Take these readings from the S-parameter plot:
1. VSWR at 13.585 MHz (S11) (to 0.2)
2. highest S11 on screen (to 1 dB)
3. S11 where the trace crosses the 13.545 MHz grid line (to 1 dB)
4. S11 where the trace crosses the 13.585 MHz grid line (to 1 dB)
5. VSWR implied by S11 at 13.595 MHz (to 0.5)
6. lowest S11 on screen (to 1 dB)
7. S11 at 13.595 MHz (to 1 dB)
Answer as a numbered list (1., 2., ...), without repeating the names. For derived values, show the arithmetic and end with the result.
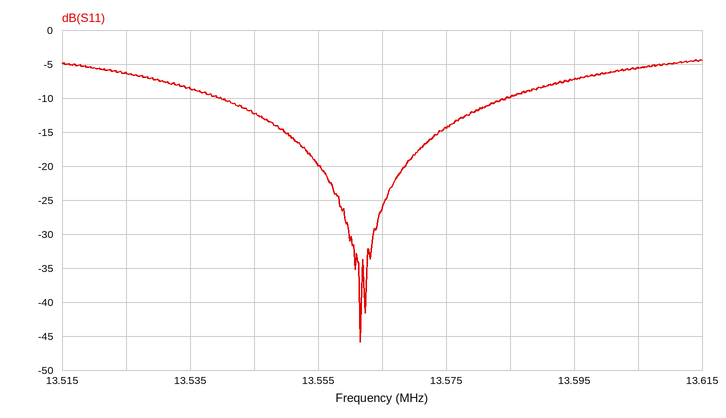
1. |Γ| = 10^(-10/20) = 0.3162; VSWR = (1 + 0.3162)/(1 − 0.3162) ≈ 1.92, so 2.0 to the nearest 0.2
2. -4 dB
3. -12 dB
4. -10 dB
5. |Γ| = 10^(-7/20) = 0.4467; VSWR = (1 + 0.4467)/(1 − 0.4467) ≈ 2.61, so 2.5 to the nearest 0.5
6. -46 dB
7. -7 dB
